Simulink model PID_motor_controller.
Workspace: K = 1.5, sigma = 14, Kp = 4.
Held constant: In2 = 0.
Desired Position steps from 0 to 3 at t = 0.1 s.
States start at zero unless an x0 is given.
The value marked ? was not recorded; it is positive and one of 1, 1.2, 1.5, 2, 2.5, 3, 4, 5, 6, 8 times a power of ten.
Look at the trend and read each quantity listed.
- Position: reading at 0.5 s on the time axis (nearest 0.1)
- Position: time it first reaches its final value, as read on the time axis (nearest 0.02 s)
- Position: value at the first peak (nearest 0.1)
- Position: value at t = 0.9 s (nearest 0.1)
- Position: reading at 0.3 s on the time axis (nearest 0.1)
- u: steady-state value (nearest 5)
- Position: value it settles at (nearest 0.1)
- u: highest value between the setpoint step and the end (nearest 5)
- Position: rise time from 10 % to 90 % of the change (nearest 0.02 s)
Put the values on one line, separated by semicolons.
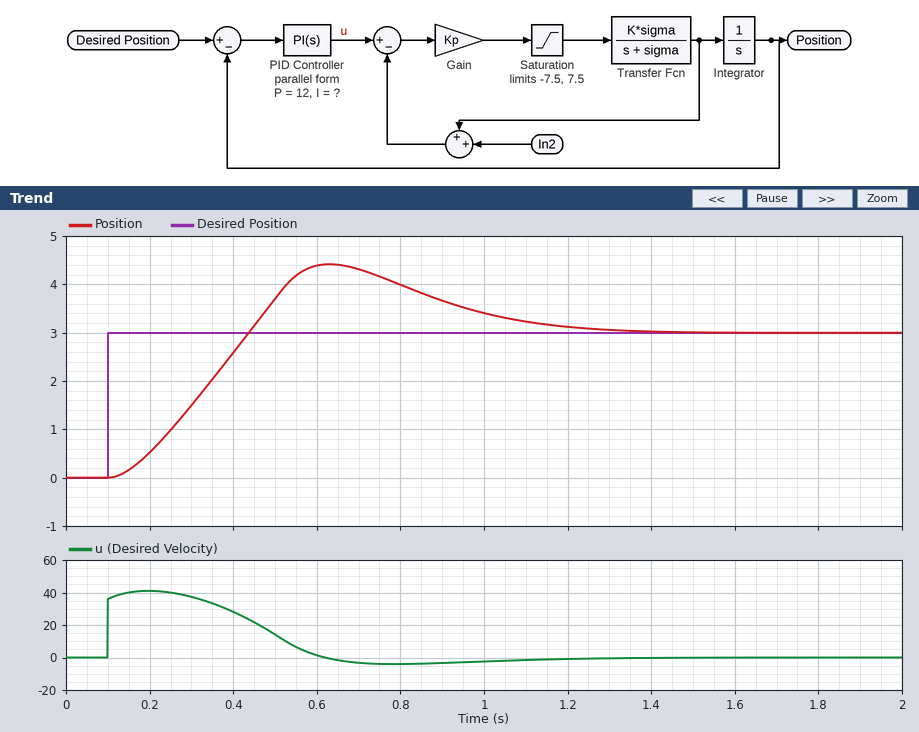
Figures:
3.7; 0.44 s; 4.4; 3.7; 1.5; 0; 3.0; 40; 0.24 s
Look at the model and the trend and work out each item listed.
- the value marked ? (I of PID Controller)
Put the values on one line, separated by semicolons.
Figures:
40
